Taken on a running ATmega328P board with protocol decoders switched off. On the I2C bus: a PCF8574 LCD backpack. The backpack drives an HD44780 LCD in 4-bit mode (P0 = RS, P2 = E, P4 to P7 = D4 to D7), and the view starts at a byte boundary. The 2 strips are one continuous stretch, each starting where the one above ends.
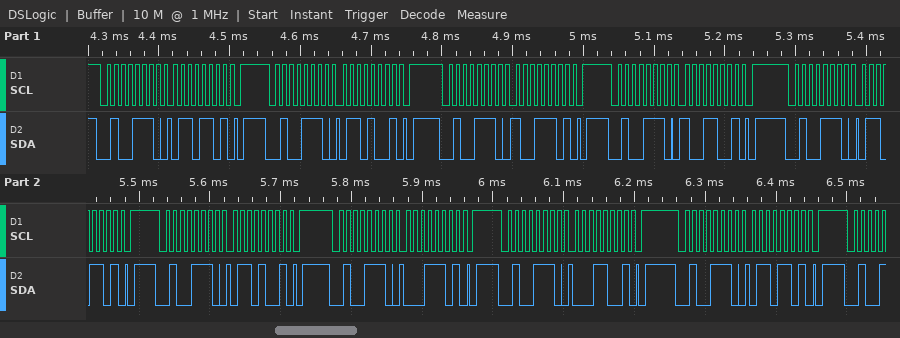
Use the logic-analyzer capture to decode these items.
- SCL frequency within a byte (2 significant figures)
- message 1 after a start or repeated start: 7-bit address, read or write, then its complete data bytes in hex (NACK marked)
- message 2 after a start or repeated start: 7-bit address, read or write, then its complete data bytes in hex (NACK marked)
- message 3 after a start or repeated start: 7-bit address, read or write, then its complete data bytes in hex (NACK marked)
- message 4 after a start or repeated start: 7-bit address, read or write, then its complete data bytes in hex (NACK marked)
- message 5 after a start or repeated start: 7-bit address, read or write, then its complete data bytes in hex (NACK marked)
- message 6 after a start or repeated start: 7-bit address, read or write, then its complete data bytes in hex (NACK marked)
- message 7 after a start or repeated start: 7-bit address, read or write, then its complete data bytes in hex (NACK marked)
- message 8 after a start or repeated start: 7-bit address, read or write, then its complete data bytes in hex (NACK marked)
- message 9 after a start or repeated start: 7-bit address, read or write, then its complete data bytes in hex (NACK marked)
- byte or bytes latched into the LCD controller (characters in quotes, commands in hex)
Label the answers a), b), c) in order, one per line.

a) 100 kHz
b) 0x27 write: 6D
c) 0x27 write: 69
d) 0x27 write: 9D
e) 0x27 write: 99
f) 0x27 write: 6D
g) 0x27 write: 69
h) 0x27 write: 1D
i) 0x27 write: 19
j) 0x27 write: 6D
k) 'i' 'a'
